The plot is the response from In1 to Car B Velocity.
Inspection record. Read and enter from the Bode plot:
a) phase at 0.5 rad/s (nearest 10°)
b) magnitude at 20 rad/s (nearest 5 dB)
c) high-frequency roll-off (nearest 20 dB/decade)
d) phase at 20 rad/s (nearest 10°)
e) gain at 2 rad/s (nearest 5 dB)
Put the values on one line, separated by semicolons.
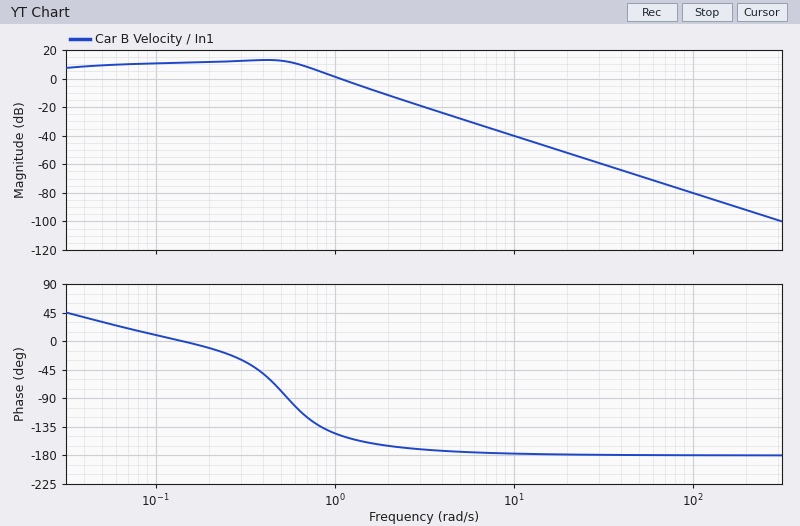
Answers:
-80°; -50 dB; -40 dB/decade; -180°; -10 dB
